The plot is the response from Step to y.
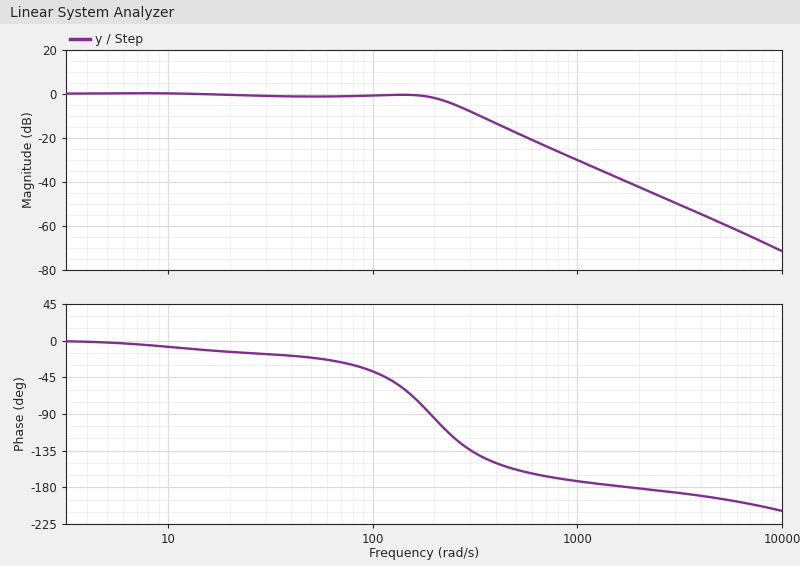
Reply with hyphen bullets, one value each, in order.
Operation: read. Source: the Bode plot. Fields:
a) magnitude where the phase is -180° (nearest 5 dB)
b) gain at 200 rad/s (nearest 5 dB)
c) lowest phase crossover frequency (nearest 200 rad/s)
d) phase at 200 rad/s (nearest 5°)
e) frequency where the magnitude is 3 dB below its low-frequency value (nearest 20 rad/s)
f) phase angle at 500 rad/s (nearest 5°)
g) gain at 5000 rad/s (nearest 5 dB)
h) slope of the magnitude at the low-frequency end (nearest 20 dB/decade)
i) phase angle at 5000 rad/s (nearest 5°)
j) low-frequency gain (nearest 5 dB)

- -40 dB
- 0 dB
- 1800 rad/s
- -95°
- 220 rad/s
- -160°
- -60 dB
- 0 dB/decade
- -195°
- 0 dB
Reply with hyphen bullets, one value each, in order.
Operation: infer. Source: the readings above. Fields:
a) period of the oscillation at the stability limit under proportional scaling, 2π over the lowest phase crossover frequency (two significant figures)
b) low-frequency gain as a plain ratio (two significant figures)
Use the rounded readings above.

- 0.0035 s
- 1.0
